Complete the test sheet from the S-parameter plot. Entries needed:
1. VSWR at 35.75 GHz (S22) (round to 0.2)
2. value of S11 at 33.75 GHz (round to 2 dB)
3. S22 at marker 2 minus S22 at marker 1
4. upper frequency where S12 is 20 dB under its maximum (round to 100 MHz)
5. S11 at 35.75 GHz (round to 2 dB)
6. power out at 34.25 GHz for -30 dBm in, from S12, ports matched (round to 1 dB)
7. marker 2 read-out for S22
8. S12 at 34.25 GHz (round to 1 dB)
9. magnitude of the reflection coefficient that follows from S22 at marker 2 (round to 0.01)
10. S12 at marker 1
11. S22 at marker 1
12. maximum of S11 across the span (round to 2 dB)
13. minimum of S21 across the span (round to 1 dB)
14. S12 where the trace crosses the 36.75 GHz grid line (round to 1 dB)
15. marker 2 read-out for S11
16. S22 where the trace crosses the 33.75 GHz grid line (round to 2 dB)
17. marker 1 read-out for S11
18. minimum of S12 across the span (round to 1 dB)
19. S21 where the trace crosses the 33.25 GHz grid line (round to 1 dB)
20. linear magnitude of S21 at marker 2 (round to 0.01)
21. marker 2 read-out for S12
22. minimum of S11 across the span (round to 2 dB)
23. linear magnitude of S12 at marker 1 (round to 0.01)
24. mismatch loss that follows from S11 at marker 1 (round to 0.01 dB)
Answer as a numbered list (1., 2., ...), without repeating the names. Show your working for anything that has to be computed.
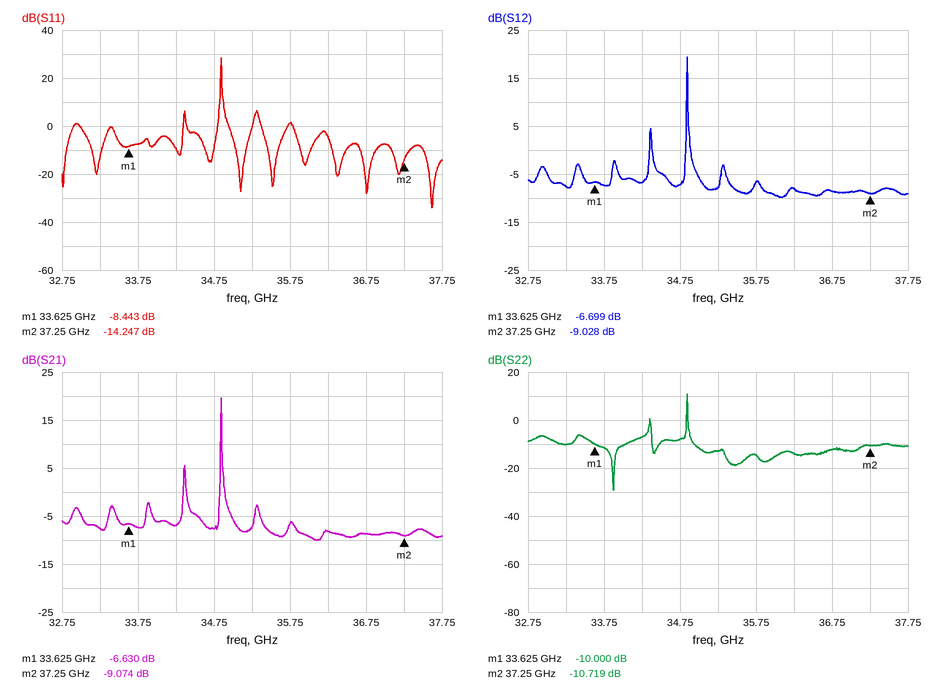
1. |Γ| = 10^(-14/20) = 0.1995; VSWR = (1 + 0.1995)/(1 − 0.1995) ≈ 1.50, so 1.4 to the nearest 0.2
2. -8 dB
3. -10.719 − (-10) = -0.719 dB
4. 34.9 GHz
5. 2 dB
6. -30 dBm + (-7 dB) = -37 dBm
7. -10.719 dB
8. -7 dB
9. 10^(-10.719/20) ≈ 0.29
10. -6.699 dB
11. -10.000 dB
12. 28 dB
13. -10 dB
14. -9 dB
15. -14.247 dB
16. -12 dB
17. -8.443 dB
18. -10 dB
19. -8 dB
20. 10^(-9.074/20) ≈ 0.35
21. -9.028 dB
22. -34 dB
23. 10^(-6.699/20) ≈ 0.46
24. −10 log10(1 − 10^(-8.443/10)) ≈ 0.67 dB
